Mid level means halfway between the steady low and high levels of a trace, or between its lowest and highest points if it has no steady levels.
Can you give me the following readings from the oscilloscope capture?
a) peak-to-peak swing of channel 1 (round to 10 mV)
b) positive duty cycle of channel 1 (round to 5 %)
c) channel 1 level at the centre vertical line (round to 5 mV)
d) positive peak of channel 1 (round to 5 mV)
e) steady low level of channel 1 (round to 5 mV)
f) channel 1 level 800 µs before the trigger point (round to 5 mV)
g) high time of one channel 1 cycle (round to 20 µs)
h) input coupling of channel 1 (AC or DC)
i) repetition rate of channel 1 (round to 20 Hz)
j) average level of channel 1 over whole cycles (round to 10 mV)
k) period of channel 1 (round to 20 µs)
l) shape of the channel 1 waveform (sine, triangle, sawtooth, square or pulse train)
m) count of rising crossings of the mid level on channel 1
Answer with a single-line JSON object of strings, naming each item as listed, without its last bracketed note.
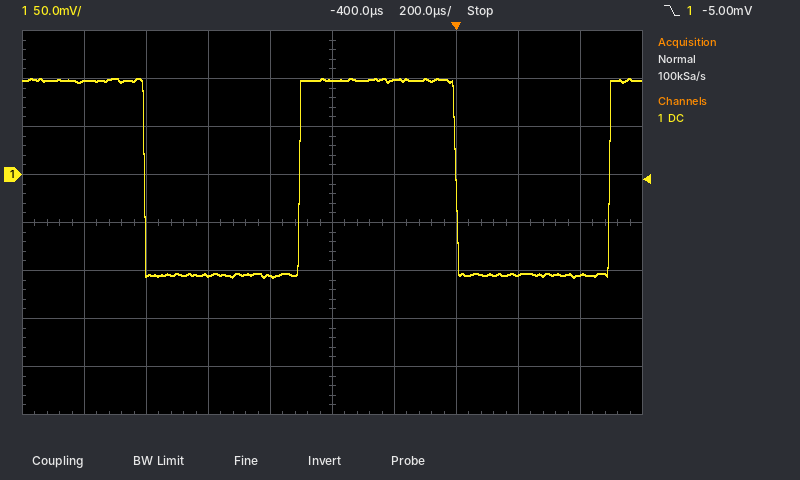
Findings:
{"peak-to-peak swing of channel 1": "210 mV", "positive duty cycle of channel 1": "50 %", "channel 1 level at the centre vertical line": "100 mV", "positive peak of channel 1": "100 mV", "steady low level of channel 1": "-105 mV", "channel 1 level 800 µs before the trigger point": "-105 mV", "high time of one channel 1 cycle": "500 µs", "input coupling of channel 1": "DC", "repetition rate of channel 1": "1.00 kHz", "average level of channel 1 over whole cycles": "0 mV", "period of channel 1": "1.00 ms", "shape of the channel 1 waveform": "square", "count of rising crossings of the mid level on channel 1": "2"}
